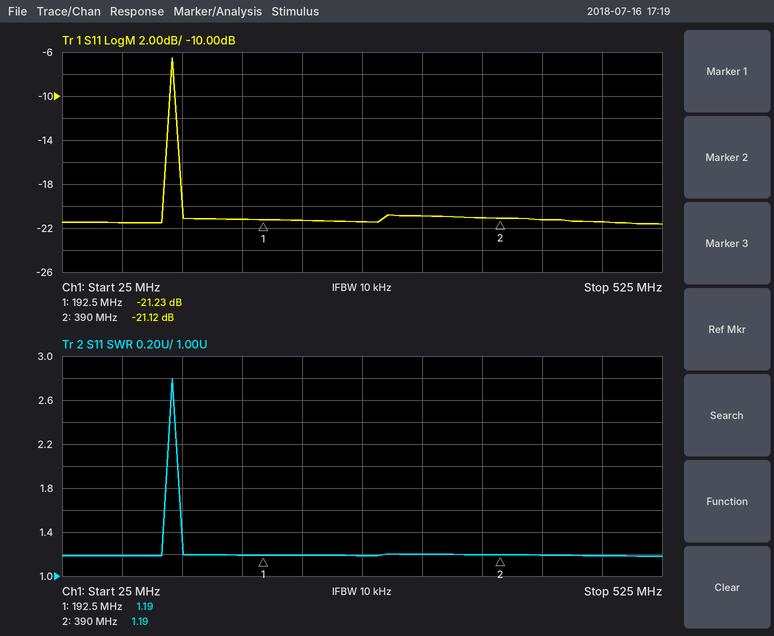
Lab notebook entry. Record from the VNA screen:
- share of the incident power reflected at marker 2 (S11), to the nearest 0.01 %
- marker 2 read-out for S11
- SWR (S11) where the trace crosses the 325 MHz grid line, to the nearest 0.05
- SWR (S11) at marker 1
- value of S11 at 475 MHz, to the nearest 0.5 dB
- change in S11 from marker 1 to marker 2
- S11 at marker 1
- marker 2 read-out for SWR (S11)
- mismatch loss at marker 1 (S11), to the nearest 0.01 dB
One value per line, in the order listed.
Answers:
0.77 %
-21.12 dB
1.20
1.19
-21.5 dB
0.11 dB
-21.23 dB
1.19
0.03 dB
